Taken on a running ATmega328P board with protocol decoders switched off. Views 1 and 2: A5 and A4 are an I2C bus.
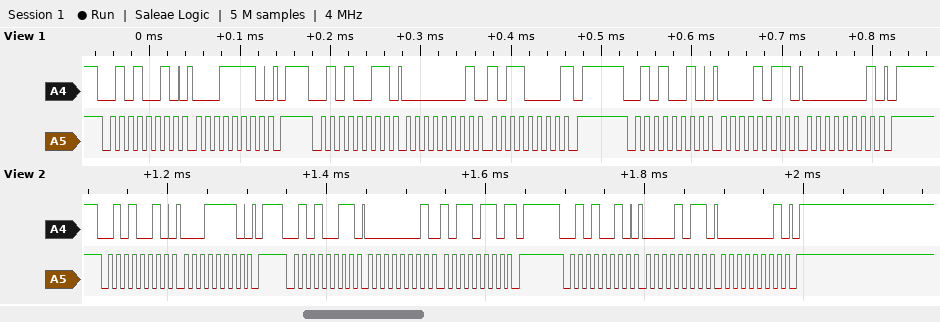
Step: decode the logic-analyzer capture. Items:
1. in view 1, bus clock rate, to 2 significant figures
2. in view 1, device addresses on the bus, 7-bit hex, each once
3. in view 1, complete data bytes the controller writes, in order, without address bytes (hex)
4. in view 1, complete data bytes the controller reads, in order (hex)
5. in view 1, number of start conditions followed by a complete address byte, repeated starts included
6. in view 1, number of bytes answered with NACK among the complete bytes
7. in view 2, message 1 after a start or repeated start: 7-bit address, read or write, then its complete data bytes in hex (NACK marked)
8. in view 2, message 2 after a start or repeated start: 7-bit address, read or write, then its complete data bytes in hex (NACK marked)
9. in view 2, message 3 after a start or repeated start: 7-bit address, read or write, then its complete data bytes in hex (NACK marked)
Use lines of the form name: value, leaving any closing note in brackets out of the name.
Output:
in view 1, bus clock rate, to 2 significant figures: 100 kHz
in view 1, device addresses on the bus, 7-bit hex, each once: 0x29
in view 1, complete data bytes the controller writes, in order, without address bytes: 1E 0B 01
in view 1, complete data bytes the controller reads, in order: 01 B0
in view 1, number of start conditions followed by a complete address byte, repeated starts included: 3
in view 1, number of bytes answered with NACK among the complete bytes: 1
in view 2, message 1 after a start or repeated start: 7-bit address, read or write, then its complete data bytes in hex: 0x29 write: 1E
in view 2, message 2 after a start or repeated start: 7-bit address, read or write, then its complete data bytes in hex: 0x29 read: 01 B6 NACK
in view 2, message 3 after a start or repeated start: 7-bit address, read or write, then its complete data bytes in hex: 0x29 write: 0B 01
